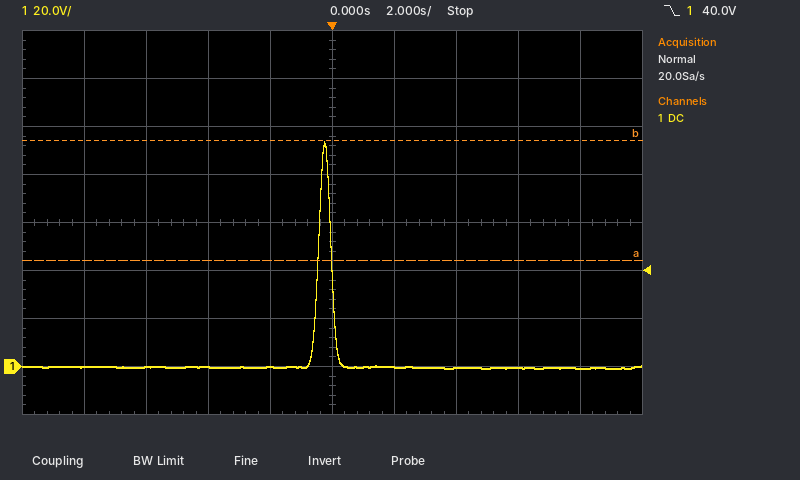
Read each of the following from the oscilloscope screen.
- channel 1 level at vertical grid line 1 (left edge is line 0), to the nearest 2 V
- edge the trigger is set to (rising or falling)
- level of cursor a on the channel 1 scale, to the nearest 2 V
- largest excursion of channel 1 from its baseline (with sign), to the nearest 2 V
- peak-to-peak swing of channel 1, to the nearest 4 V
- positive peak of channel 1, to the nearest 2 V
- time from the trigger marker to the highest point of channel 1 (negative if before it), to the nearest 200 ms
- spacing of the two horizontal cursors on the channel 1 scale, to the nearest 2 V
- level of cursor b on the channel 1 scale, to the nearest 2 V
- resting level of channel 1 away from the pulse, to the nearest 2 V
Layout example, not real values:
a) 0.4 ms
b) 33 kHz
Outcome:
a) 0 V
b) falling
c) 44 V
d) +94 V
e) 96 V
f) 94 V
g) -200 ms
h) 50 V
i) 94 V
j) 0 V
